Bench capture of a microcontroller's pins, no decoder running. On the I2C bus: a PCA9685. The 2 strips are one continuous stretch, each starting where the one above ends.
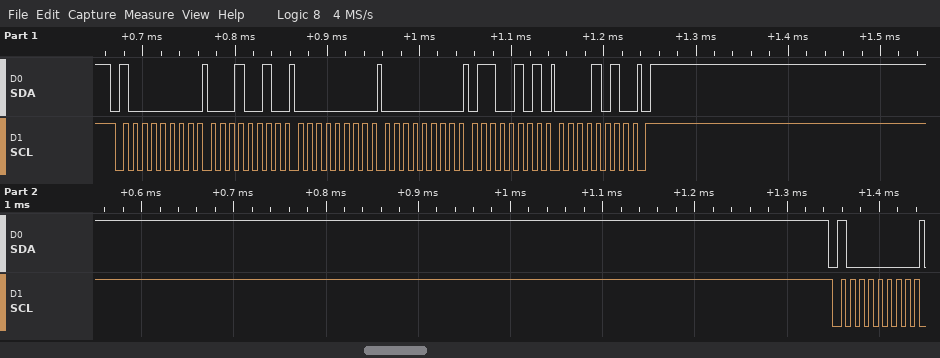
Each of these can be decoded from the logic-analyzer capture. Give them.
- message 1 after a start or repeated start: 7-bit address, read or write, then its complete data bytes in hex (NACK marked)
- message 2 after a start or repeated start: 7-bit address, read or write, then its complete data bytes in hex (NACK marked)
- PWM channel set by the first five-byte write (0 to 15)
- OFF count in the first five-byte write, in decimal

0x40 write: 12 00 00 65 0A
0x40 write
3
2661
